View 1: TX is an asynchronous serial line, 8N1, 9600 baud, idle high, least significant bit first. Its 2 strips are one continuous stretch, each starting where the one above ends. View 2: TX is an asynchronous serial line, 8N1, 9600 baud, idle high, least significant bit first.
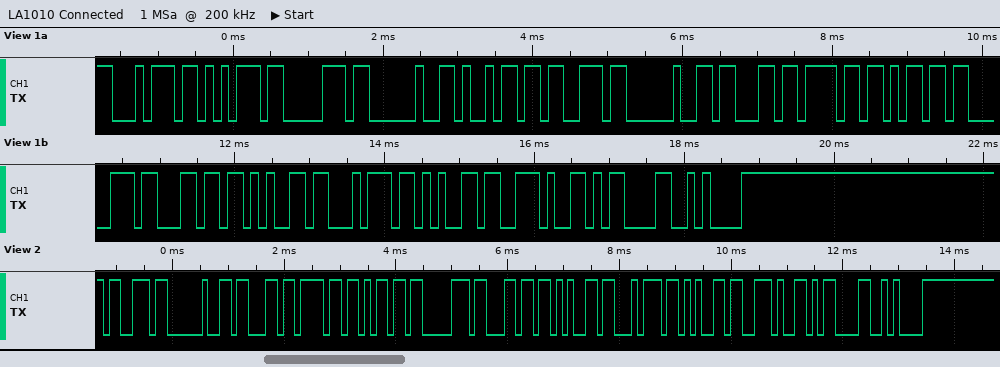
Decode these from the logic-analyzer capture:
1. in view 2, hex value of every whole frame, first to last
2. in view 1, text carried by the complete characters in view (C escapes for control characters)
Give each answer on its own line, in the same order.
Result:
0x73 0x20 0x63 0x6F 0x6D 0x70 0x6C 0x65 0x74 0x65 0x2E 0x0D 0x0A
"tup is complete.\r\n"
